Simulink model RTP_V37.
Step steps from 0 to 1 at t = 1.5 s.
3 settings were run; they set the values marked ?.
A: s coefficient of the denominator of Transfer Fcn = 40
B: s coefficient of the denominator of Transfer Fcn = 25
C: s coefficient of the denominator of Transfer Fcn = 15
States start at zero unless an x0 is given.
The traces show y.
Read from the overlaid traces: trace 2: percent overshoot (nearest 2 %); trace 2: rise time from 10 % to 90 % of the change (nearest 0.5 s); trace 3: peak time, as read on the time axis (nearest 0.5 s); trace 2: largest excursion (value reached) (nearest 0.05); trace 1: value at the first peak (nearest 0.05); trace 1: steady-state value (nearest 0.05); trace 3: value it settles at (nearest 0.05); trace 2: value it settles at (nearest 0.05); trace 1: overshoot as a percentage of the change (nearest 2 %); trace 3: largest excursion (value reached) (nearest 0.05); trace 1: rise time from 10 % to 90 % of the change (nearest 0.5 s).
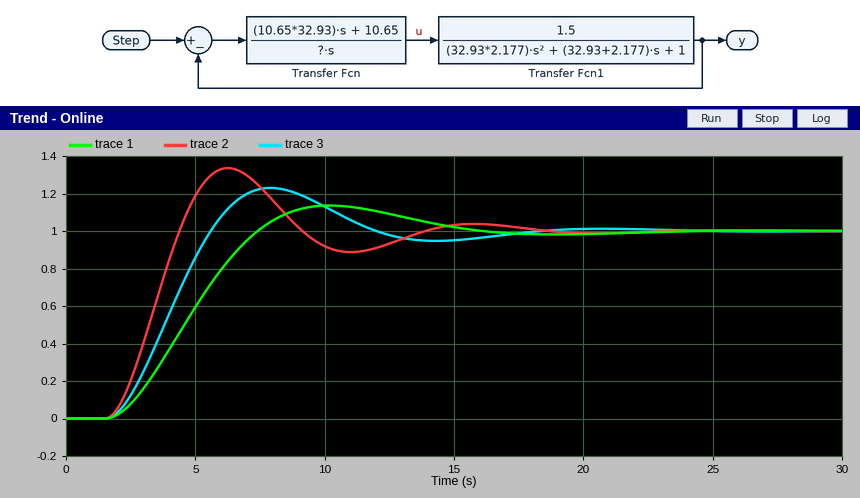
34 %
2.0 s
8.0 s
1.35
1.15
1.00
1.00
1.00
14 %
1.25
4.0 s
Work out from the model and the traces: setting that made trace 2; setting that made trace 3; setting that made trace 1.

C
B
A
